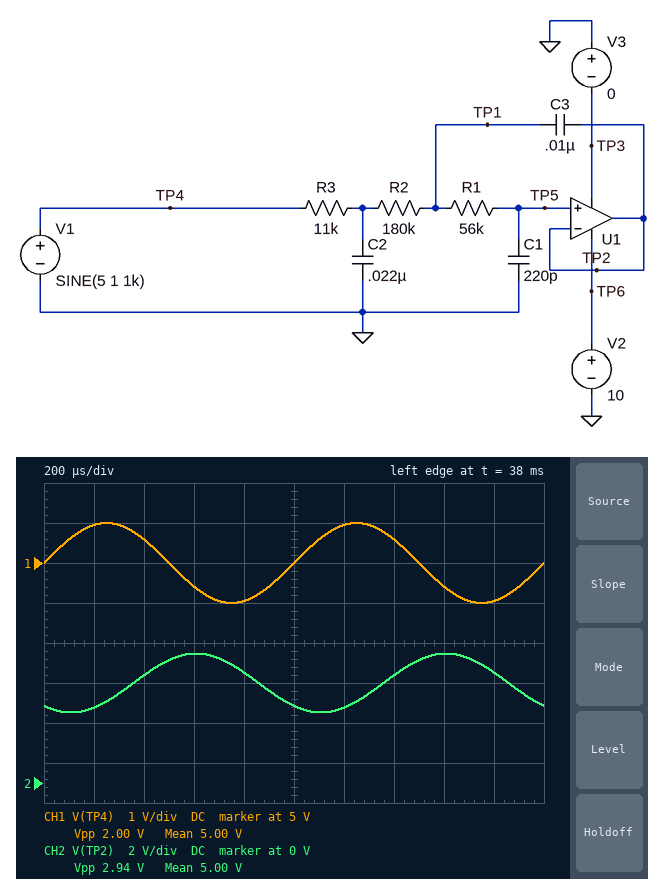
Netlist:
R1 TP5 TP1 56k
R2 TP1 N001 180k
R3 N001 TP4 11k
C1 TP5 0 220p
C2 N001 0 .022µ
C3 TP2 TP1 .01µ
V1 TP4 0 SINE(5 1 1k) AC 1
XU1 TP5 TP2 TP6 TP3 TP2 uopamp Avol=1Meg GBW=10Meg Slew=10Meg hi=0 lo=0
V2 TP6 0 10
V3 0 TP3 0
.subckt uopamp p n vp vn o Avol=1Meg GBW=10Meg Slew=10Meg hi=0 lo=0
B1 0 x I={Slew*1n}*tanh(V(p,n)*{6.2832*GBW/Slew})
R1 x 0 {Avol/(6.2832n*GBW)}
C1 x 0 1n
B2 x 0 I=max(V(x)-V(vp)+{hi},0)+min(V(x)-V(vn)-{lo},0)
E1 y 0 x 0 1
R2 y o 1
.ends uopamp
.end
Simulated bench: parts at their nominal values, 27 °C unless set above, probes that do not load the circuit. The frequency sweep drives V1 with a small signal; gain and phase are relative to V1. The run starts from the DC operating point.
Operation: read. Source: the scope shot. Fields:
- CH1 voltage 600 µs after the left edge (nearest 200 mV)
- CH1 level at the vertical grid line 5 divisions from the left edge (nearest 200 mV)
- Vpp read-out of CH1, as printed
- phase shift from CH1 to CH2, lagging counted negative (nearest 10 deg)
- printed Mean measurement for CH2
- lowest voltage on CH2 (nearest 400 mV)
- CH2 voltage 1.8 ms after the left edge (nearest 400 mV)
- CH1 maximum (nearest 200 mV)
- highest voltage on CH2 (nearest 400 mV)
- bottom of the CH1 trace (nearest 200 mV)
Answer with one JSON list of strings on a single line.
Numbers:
["4.4 V", "5.0 V", "2.00 V", "-130 deg", "5.00 V", "3.6 V", "5.6 V", "6.0 V", "6.4 V", "4.0 V"]
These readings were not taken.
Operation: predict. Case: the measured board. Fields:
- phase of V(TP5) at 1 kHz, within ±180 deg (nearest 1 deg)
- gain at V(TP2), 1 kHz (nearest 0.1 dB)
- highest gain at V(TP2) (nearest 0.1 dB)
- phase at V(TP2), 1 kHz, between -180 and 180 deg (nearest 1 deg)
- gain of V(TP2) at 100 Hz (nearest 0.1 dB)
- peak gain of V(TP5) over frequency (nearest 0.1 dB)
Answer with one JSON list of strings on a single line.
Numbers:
["-129 deg", "3.4 dB", "3.4 dB", "-129 deg", "0 dB", "3.4 dB"]
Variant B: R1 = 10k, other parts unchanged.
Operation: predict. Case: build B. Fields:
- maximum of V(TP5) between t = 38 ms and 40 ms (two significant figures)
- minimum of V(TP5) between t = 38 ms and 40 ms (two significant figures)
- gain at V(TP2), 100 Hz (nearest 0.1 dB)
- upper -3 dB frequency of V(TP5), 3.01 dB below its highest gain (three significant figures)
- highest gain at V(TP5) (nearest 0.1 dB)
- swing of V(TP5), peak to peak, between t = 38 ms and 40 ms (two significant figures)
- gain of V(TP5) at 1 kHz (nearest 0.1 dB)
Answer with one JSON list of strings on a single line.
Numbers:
["5.6 V", "4.4 V", "-0.1 dB", "741 Hz", "0 dB", "1.2 V", "-4.2 dB"]
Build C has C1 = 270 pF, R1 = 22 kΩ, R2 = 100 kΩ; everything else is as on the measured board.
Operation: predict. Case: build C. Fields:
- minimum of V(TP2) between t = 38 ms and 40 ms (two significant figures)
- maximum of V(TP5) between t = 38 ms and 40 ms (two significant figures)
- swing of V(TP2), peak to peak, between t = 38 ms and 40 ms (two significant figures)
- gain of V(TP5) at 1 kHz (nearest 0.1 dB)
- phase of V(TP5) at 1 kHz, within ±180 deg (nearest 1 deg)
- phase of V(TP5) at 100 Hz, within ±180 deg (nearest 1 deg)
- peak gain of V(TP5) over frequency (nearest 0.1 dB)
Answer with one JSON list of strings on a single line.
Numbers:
["4.3 V", "5.7 V", "1.4 V", "-3.2 dB", "-73 deg", "-10 deg", "0 dB"]
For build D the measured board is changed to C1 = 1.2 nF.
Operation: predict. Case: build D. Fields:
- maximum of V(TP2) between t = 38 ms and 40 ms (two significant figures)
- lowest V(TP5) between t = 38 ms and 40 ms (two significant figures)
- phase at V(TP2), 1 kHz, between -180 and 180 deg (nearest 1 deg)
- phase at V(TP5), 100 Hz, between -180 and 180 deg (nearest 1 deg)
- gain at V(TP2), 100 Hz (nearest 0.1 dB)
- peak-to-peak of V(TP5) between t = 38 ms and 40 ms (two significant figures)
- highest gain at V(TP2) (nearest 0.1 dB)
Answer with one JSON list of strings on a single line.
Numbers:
["5.1 V", "4.9 V", "150 deg", "-20 deg", "0.2 dB", "260 mV", "1.2 dB"]
